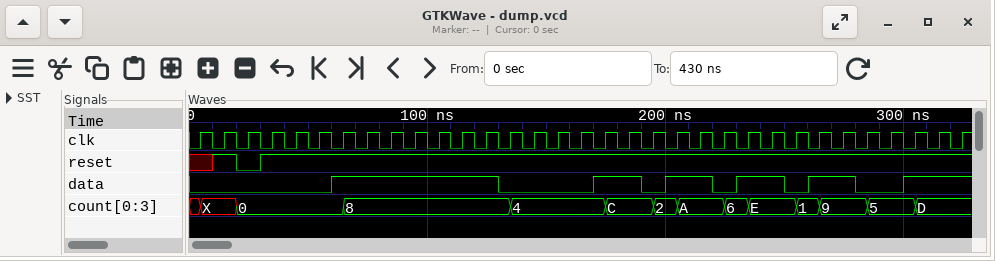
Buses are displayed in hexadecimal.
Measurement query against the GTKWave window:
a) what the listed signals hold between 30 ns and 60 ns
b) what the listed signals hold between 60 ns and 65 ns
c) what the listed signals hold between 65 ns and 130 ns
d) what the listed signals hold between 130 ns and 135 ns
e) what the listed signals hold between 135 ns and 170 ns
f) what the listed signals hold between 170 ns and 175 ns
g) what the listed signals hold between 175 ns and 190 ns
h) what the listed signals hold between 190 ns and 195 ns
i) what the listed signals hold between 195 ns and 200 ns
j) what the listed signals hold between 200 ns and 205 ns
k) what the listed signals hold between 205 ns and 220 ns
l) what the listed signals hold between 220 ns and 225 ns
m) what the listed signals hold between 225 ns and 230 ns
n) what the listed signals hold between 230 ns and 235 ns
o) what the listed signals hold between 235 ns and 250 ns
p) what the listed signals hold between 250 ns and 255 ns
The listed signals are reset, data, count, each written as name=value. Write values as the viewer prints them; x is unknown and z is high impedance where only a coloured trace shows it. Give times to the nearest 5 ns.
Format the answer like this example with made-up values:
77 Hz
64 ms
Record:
reset=1, data=0, count=0
reset=1, data=1, count=0
reset=1, data=1, count=8
reset=1, data=0, count=8
reset=1, data=0, count=4
reset=1, data=1, count=4
reset=1, data=1, count=C
reset=1, data=0, count=C
reset=1, data=0, count=2
reset=1, data=1, count=2
reset=1, data=1, count=A
reset=1, data=0, count=A
reset=1, data=0, count=6
reset=1, data=1, count=6
reset=1, data=1, count=E
reset=1, data=0, count=E
